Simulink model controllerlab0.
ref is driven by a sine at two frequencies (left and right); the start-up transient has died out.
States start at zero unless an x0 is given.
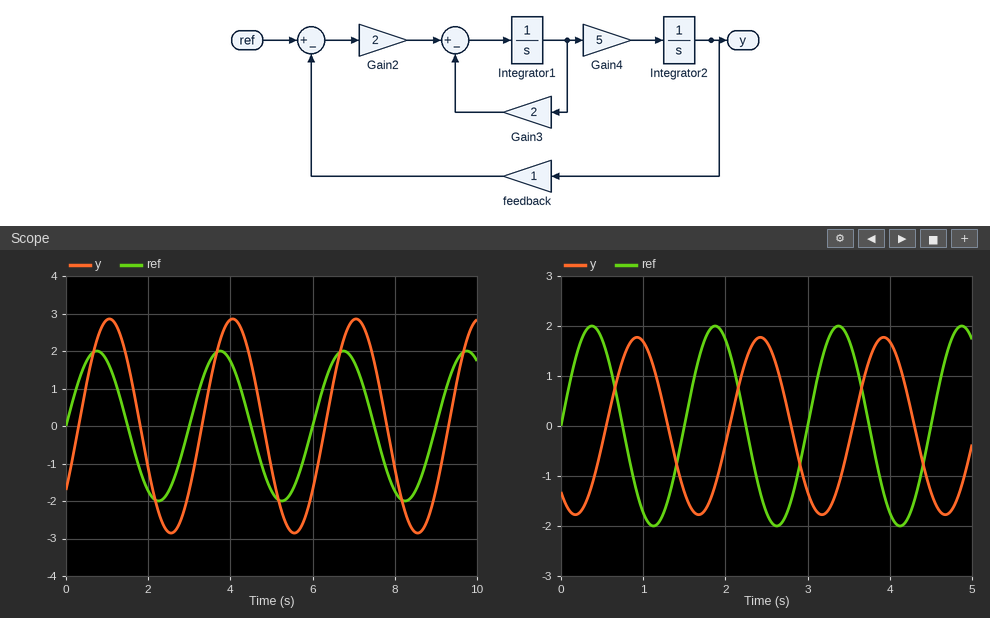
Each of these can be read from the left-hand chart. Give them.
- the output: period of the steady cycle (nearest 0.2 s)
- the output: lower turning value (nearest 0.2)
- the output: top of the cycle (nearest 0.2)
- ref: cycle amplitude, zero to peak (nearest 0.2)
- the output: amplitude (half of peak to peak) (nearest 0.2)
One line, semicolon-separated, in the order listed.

3.0 s; -2.8; 2.8; 2.0; 2.8
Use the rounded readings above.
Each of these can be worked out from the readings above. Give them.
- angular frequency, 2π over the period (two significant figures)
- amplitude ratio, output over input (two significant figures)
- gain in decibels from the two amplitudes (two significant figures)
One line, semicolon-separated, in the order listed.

2.1 rad/s; 1.4; 2.9 dB
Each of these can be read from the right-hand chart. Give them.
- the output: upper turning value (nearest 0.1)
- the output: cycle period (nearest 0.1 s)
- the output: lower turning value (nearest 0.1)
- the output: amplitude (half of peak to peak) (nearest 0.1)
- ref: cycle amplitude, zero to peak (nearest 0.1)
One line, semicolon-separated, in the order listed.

1.8; 1.5 s; -1.8; 1.8; 2.0
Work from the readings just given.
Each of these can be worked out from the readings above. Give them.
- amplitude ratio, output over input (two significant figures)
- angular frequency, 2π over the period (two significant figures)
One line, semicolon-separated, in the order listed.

0.90; 4.2 rad/s
